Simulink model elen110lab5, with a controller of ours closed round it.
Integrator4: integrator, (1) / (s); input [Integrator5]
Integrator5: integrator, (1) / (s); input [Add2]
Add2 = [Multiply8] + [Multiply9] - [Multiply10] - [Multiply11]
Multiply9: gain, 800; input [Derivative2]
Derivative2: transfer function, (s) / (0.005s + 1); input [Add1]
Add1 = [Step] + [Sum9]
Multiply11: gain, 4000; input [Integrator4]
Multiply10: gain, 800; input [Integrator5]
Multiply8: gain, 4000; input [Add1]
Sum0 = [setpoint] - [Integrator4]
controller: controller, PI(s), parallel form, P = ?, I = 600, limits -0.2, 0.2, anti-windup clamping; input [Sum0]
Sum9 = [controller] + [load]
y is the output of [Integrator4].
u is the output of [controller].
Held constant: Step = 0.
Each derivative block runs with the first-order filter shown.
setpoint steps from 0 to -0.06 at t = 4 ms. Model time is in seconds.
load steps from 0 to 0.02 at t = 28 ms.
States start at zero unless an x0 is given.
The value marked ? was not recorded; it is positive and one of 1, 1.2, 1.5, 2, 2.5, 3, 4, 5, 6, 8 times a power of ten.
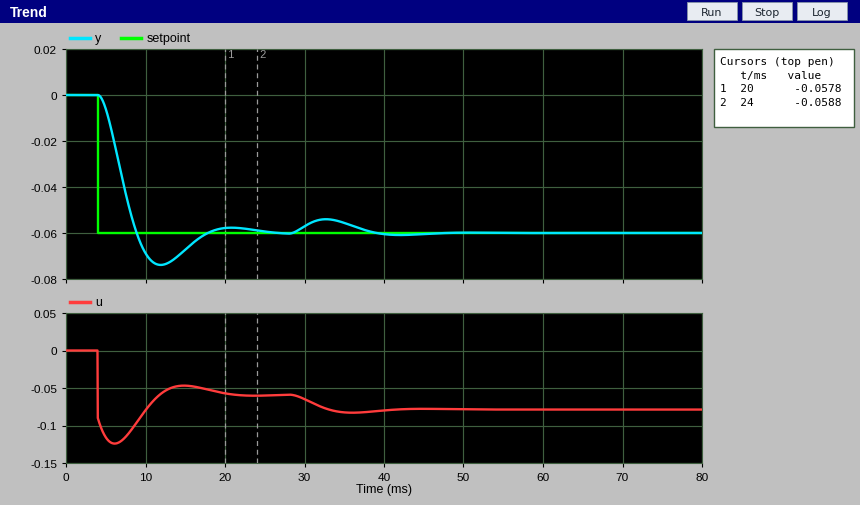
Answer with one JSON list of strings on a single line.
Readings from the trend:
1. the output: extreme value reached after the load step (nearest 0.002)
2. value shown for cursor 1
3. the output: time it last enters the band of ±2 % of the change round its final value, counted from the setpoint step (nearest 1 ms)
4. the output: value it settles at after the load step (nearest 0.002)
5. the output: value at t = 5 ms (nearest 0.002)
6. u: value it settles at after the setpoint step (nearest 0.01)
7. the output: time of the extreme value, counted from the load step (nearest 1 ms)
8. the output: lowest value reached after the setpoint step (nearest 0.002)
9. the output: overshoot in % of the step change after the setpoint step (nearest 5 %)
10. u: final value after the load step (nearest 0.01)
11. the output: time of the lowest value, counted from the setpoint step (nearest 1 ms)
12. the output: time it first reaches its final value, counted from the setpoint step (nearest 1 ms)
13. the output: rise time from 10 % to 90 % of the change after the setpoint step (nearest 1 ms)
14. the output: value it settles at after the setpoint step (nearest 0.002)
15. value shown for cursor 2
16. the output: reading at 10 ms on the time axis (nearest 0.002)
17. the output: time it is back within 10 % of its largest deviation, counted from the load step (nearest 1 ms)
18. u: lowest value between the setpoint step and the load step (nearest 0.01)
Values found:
["-0.054", "-0.0578", "20 ms", "-0.060", "-0.006", "-0.06", "5 ms", "-0.074", "25 %", "-0.08", "8 ms", "5 ms", "3 ms", "-0.060", "-0.0588", "-0.068", "16 ms", "-0.12"]
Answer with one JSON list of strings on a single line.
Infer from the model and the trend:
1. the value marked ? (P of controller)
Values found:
["1.5"]
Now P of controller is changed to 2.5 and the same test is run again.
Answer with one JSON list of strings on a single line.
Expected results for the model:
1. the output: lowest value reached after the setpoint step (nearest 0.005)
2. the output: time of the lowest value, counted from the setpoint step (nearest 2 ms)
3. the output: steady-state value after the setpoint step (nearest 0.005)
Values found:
["-0.070", "6 ms", "-0.060"]
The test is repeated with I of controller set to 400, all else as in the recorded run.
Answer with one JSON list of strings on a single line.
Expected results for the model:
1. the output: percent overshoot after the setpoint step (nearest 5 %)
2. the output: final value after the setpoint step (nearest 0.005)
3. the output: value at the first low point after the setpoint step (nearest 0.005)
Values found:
["10 %", "-0.060", "-0.065"]
